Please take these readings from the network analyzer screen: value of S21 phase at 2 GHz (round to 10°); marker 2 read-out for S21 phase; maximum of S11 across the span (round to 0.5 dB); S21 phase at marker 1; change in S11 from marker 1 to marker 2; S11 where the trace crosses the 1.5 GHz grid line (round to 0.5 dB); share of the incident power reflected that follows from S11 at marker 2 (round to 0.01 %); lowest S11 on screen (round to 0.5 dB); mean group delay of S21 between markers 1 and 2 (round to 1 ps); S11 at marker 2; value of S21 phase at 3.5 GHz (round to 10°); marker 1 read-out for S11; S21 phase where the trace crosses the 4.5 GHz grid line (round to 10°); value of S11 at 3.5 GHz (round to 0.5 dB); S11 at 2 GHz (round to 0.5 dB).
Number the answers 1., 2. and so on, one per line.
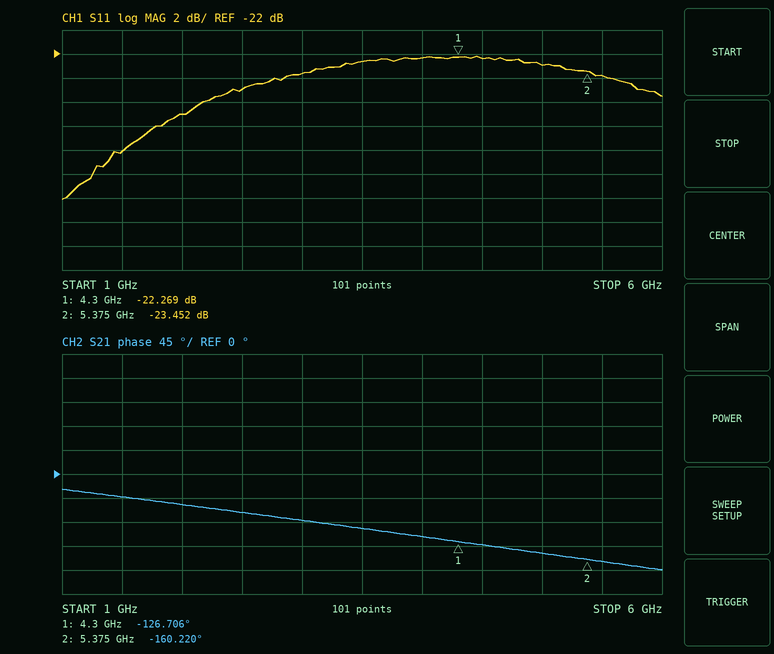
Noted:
1. -60°
2. -160.220°
3. -22.0 dB
4. -126.706°
5. -1.183 dB
6. -30.0 dB
7. 0.45 %
8. -34.0 dB
9. 87 ps
10. -23.452 dB
11. -100°
12. -22.269 dB
13. -130°
14. -22.5 dB
15. -27.0 dB
